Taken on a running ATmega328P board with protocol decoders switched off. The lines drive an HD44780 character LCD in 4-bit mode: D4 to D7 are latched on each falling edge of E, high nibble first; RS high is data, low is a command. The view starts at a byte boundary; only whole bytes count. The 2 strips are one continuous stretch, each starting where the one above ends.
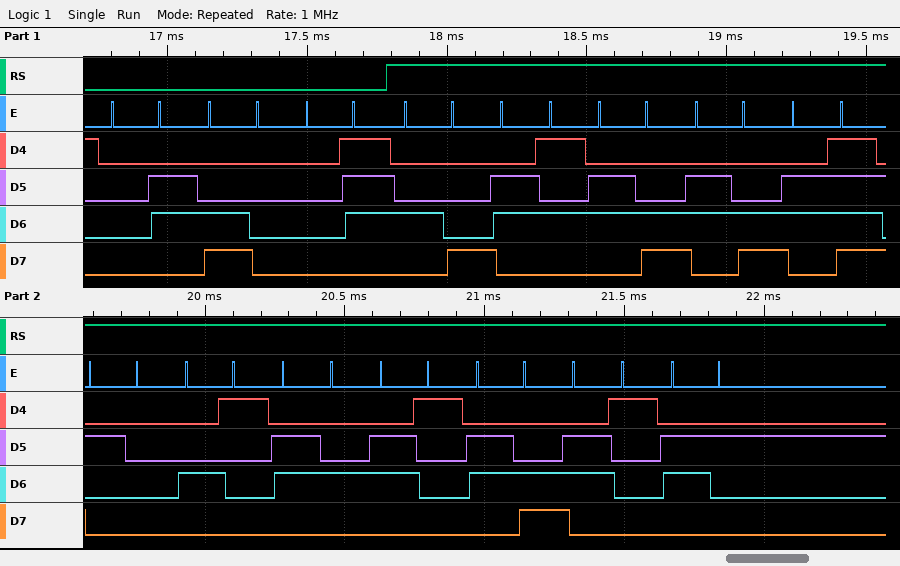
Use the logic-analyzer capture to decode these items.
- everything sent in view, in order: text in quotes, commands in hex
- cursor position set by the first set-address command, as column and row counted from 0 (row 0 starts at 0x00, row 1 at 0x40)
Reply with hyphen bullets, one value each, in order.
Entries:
- 0x06 0xC0 0x07 "Hello Adalab"
- column 0, row 1
